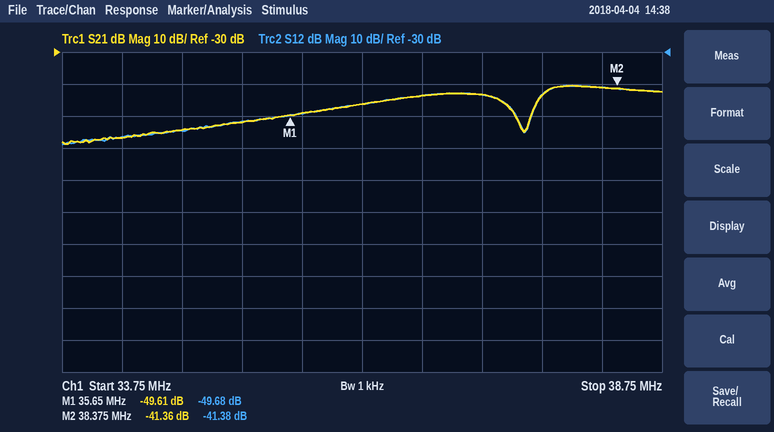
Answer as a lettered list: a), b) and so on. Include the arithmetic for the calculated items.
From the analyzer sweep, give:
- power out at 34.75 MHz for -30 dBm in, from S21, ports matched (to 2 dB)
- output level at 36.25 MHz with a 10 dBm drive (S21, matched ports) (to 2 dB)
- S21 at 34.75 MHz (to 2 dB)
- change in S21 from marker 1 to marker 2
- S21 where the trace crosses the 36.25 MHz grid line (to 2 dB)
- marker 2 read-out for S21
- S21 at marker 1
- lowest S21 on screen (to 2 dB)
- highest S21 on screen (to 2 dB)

a) -30 dBm + (-54 dB) = -84 dBm
b) 10 dBm + (-46 dB) = -36 dBm
c) -54 dB
d) -41.36 − (-49.61) = 8.25 dB
e) -46 dB
f) -41.36 dB
g) -49.61 dB
h) -58 dB
i) -40 dB
